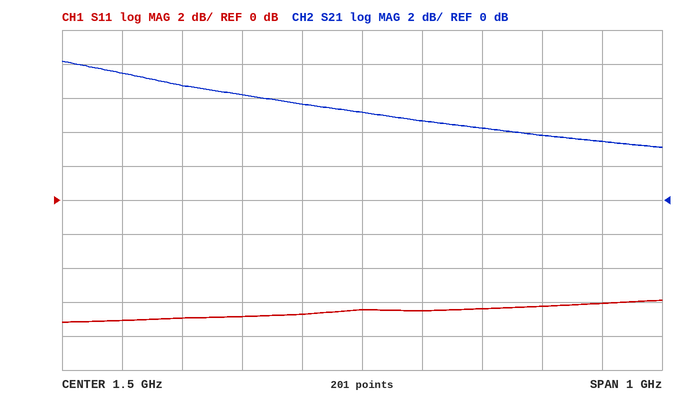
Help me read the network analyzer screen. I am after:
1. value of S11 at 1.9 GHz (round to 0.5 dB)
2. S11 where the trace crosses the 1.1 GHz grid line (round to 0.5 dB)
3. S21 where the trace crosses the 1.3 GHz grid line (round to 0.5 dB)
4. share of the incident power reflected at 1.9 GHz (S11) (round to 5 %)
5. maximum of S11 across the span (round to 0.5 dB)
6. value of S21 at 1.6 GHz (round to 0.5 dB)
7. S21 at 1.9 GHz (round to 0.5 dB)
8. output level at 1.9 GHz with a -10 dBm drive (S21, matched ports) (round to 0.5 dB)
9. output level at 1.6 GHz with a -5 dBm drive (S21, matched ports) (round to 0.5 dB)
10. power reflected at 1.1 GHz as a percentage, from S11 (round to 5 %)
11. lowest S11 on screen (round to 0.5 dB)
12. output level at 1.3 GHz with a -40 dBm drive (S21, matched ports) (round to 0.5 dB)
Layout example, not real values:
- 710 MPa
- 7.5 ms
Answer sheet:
- -6.0 dB
- -7.0 dB
- 6.0 dB
- 25 %
- -6.0 dB
- 4.5 dB
- 3.5 dB
- -6.5 dBm
- -0.5 dBm
- 20 %
- -7.0 dB
- -34.0 dBm
